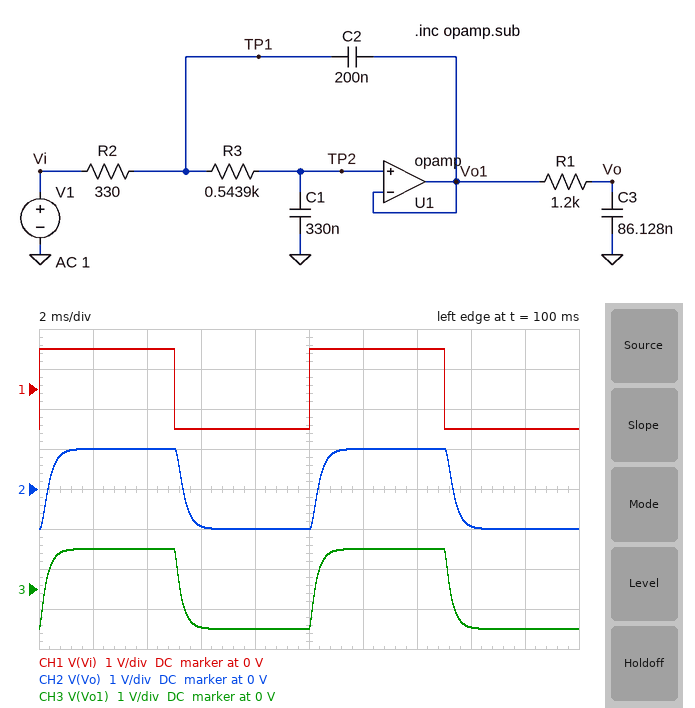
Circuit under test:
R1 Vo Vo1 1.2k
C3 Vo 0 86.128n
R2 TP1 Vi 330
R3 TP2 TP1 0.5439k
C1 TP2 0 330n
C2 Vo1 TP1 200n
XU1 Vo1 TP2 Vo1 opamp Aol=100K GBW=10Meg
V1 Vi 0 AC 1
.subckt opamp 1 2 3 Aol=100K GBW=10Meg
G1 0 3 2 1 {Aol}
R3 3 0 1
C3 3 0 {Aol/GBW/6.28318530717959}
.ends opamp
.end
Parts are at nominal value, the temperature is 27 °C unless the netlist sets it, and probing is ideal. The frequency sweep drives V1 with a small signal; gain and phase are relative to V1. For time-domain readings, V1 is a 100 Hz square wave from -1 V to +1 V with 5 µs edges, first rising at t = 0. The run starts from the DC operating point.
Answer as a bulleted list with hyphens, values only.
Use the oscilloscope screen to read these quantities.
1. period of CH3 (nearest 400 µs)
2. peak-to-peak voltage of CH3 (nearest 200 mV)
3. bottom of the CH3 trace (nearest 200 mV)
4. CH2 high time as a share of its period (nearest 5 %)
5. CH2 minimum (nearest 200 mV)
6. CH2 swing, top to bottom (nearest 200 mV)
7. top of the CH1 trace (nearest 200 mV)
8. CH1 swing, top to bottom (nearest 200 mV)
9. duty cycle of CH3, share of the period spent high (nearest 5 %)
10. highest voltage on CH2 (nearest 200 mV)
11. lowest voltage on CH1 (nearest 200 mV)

- 10.0 ms
- 2.0 V
- -1.0 V
- 50 %
- -1.0 V
- 2.0 V
- 1.0 V
- 2.0 V
- 50 %
- 1.0 V
- -1.0 V
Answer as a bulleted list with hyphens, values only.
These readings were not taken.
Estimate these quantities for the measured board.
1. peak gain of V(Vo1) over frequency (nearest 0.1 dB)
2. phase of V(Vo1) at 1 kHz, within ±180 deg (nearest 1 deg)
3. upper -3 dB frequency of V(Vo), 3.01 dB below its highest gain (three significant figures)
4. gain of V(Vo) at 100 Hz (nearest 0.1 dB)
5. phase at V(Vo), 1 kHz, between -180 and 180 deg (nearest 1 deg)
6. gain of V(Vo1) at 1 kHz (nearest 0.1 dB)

- 0 dB
- -74 deg
- 562 Hz
- -0.1 dB
- -107 deg
- -5.5 dB
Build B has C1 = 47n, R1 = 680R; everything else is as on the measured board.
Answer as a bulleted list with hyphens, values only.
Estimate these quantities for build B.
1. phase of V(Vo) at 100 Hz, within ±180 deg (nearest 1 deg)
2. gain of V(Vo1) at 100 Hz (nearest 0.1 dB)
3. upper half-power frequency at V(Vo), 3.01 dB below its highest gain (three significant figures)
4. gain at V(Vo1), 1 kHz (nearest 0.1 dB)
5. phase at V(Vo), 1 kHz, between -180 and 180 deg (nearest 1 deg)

- -4 deg
- 0 dB
- 3.32 kHz
- 0.3 dB
- -36 deg
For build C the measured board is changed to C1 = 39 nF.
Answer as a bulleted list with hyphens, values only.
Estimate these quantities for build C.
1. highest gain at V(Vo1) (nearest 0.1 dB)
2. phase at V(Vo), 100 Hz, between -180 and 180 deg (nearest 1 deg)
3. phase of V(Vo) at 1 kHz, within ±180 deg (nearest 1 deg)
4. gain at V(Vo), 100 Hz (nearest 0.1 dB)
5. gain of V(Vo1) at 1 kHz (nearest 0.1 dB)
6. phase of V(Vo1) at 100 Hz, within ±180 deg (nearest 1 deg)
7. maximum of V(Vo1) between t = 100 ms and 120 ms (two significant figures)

- 1.8 dB
- -5 deg
- -46 deg
- 0 dB
- 0.3 dB
- -1 deg
- 1.4 V
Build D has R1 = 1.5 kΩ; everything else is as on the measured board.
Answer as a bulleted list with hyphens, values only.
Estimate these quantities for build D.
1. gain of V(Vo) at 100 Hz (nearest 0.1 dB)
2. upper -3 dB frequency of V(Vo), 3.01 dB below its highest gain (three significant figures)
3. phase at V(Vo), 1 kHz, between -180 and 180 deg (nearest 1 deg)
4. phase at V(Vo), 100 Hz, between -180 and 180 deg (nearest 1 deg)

- -0.1 dB
- 533 Hz
- -113 deg
- -15 deg
